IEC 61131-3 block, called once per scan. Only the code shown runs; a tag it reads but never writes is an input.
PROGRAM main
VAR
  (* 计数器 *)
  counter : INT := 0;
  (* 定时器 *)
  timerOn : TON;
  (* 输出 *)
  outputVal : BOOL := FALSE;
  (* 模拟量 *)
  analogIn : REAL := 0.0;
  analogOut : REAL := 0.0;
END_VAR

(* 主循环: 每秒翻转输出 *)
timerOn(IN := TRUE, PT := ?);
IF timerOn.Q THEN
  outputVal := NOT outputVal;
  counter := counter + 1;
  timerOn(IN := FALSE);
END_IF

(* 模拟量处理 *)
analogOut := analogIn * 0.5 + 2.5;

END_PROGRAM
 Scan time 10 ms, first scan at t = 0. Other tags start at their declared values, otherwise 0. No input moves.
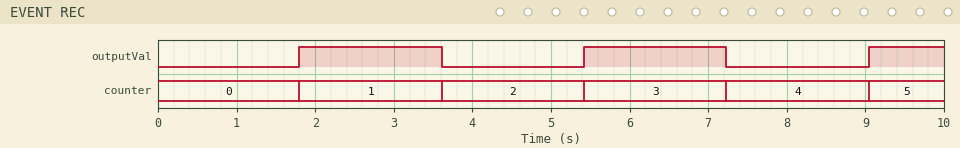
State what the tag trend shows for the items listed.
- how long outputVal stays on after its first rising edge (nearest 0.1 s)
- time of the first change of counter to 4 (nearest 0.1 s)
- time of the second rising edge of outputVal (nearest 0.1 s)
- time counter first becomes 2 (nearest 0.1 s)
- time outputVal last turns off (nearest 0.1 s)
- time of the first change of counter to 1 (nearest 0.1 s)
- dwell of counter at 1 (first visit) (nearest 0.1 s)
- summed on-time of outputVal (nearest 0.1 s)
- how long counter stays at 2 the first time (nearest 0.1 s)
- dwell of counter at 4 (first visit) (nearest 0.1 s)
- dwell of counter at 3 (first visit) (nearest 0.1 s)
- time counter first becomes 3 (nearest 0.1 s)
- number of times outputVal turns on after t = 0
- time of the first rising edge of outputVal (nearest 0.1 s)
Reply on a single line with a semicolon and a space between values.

1.8 s; 7.2 s; 5.4 s; 3.6 s; 7.2 s; 1.8 s; 1.8 s; 4.6 s; 1.8 s; 1.8 s; 1.8 s; 5.4 s; 3; 1.8 s
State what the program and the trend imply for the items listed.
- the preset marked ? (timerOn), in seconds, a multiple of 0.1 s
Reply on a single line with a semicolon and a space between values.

1.8 s
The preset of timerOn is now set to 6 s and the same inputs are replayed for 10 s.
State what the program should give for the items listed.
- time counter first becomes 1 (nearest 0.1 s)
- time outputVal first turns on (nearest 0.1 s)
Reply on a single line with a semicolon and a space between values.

6.0 s; 6.0 s
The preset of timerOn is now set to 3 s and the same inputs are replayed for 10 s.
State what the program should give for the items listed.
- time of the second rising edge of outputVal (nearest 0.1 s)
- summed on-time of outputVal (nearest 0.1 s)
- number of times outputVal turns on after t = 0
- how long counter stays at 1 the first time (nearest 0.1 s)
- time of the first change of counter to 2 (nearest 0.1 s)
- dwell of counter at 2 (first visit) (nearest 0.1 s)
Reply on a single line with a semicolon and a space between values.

9.0 s; 4.0 s; 2; 3.0 s; 6.0 s; 3.0 s
